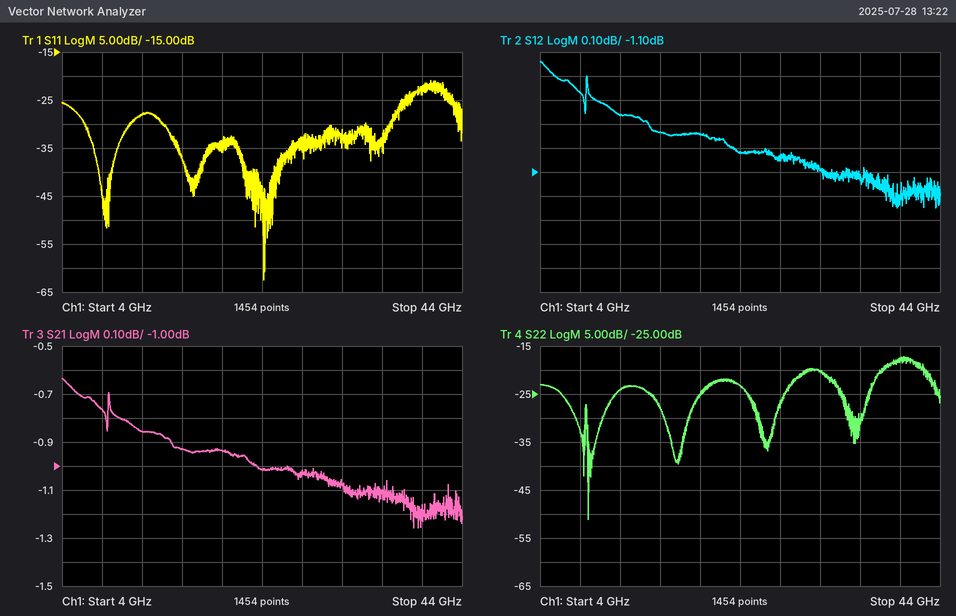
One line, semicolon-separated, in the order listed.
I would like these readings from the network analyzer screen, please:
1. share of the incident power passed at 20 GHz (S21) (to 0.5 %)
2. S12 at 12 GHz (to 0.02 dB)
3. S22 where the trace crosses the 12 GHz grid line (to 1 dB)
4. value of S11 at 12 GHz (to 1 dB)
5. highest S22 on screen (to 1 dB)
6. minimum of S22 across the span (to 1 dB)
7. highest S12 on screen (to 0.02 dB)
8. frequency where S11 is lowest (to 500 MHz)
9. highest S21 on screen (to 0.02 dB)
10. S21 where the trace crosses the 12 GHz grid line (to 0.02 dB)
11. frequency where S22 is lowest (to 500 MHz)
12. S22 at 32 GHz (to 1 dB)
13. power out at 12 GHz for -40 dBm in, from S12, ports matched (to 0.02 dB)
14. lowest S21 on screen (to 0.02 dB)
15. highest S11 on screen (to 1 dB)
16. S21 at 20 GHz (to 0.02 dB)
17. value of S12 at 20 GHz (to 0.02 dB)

80.5 %; -0.86 dB; -24 dB; -28 dB; -17 dB; -51 dB; -0.64 dB; 24.0 GHz; -0.64 dB; -0.86 dB; 9.0 GHz; -20 dB; -40.86 dBm; -1.26 dB; -21 dB; -0.94 dB; -0.94 dB
